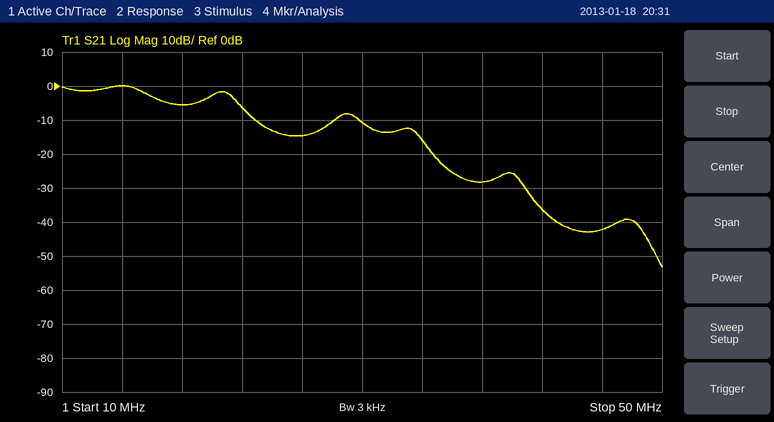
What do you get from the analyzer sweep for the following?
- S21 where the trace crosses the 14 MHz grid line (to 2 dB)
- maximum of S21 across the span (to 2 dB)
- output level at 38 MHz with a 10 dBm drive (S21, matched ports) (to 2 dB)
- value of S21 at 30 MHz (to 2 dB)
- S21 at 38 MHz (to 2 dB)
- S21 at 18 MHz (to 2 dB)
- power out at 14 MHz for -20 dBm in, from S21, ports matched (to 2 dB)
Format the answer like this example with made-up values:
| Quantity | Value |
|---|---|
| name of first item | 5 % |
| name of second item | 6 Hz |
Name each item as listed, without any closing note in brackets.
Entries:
| Quantity | Value |
|---|---|
| S21 where the trace crosses the 14 MHz grid line | 0 dB |
| maximum of S21 across the span | 0 dB |
| output level at 38 MHz with a 10 dBm drive (S21, matched ports) | -18 dBm |
| value of S21 at 30 MHz | -10 dB |
| S21 at 38 MHz | -28 dB |
| S21 at 18 MHz | -6 dB |
| power out at 14 MHz for -20 dBm in, from S21, ports matched | -20 dBm |
